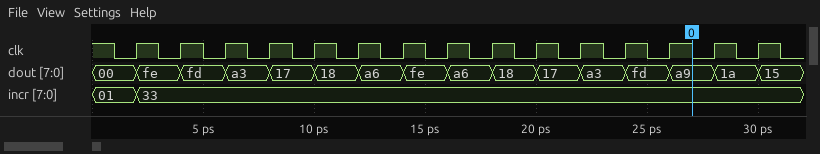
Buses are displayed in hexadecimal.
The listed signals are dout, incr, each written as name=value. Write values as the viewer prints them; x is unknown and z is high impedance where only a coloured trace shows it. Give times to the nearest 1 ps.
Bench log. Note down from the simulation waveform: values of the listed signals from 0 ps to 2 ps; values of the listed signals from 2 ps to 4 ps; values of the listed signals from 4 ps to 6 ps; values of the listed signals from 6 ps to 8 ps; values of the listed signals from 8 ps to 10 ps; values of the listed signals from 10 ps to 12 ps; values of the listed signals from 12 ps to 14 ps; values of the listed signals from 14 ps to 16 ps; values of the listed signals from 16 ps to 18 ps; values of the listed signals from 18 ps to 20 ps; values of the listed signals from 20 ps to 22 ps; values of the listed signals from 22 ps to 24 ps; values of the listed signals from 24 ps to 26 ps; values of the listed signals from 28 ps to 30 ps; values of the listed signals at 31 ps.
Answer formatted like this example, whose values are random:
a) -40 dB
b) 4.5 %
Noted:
a) dout=00, incr=01
b) dout=fe, incr=33
c) dout=fd, incr=33
d) dout=a3, incr=33
e) dout=17, incr=33
f) dout=18, incr=33
g) dout=a6, incr=33
h) dout=fe, incr=33
i) dout=a6, incr=33
j) dout=18, incr=33
k) dout=17, incr=33
l) dout=a3, incr=33
m) dout=fd, incr=33
n) dout=1a, incr=33
o) dout=15, incr=33
